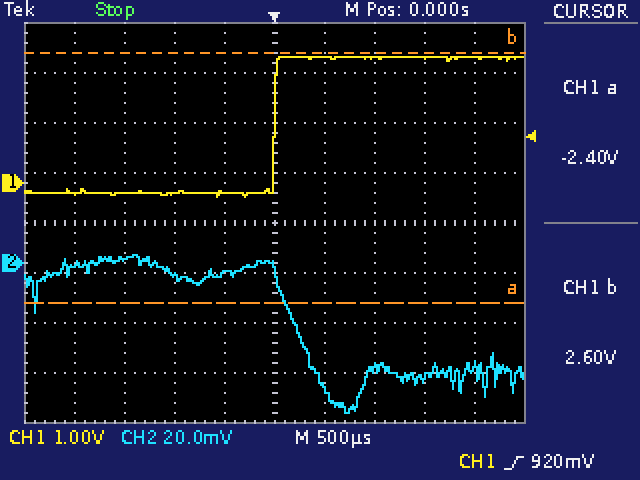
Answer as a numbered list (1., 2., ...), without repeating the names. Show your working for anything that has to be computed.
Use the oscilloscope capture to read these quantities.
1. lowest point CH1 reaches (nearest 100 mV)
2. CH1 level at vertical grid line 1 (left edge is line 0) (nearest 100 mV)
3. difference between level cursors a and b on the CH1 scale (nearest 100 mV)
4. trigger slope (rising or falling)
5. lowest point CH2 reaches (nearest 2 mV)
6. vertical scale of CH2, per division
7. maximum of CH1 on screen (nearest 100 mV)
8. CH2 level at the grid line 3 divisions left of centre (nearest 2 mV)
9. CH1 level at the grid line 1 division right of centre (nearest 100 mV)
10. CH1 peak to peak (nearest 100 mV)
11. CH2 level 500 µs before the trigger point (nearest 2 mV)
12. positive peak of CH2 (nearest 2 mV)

1. -300 mV
2. -200 mV
3. 5.0 V
4. rising
5. -60 mV
6. 20 mV
7. 2.5 V
8. 2 mV
9. 2.5 V
10. 2.5 V − (-300 mV) = 2.8 V
11. -4 mV
12. 4 mV
